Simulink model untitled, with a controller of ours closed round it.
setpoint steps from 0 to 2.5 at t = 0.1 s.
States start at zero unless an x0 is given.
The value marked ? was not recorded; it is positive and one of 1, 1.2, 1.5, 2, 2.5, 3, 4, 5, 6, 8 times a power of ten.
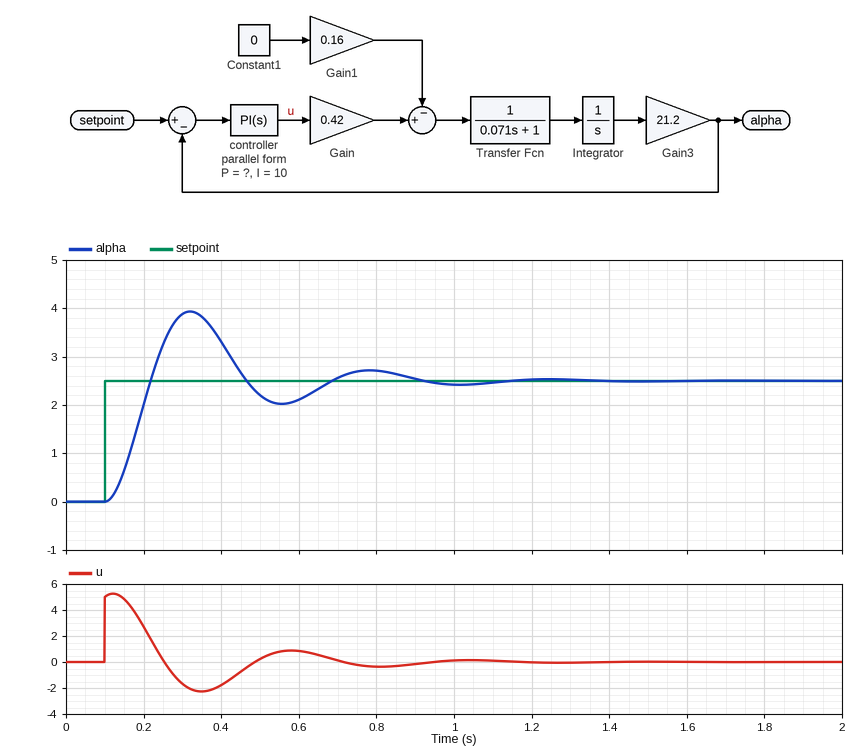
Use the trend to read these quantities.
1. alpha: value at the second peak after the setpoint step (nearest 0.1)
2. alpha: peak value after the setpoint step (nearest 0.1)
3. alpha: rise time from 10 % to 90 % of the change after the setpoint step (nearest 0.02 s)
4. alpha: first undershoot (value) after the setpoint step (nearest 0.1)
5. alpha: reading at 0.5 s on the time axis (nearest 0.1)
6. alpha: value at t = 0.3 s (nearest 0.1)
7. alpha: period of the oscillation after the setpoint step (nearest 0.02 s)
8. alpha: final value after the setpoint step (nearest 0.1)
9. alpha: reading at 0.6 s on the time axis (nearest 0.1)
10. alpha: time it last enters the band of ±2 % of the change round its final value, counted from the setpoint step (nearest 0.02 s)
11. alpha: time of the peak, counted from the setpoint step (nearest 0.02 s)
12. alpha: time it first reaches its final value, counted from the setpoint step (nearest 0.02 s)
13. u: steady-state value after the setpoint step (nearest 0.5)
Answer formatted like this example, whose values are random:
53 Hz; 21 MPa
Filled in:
2.7; 3.9; 0.08 s; 2.0; 2.2; 3.9; 0.46 s; 2.5; 2.1; 0.98 s; 0.22 s; 0.12 s; 0.0
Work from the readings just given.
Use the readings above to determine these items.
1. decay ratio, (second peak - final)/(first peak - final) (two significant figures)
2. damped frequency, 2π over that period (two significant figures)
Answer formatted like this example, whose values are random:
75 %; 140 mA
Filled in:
0.14; 14 rad/s
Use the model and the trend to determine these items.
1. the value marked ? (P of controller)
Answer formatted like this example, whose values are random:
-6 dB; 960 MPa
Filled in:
2
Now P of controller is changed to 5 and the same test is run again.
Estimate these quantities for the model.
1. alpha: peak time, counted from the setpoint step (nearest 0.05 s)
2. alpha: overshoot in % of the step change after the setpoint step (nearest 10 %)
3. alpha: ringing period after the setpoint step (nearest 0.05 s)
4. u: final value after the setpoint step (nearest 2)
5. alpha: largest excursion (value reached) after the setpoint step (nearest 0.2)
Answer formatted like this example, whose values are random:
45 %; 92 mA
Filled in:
0.15 s; 50 %; 0.25 s; 0; 3.8
